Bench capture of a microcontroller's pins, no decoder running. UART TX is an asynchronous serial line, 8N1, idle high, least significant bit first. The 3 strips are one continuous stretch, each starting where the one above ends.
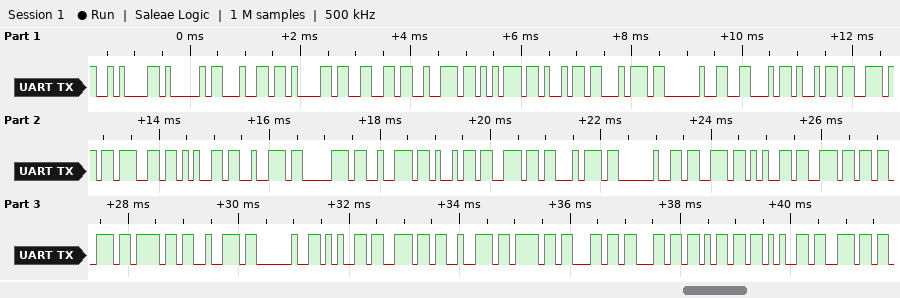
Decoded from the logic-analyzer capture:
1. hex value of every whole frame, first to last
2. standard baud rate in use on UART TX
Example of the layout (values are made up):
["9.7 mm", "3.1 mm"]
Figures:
["0A 41 64 61 66 72 75 69 74 20 46 69 6E 67 65 72 70 72 69 6E 74 20 73 65 6E 73 6F 72 20 65 6E 72 6F 6C 6C 6D 65 6E", "9600 baud"]
